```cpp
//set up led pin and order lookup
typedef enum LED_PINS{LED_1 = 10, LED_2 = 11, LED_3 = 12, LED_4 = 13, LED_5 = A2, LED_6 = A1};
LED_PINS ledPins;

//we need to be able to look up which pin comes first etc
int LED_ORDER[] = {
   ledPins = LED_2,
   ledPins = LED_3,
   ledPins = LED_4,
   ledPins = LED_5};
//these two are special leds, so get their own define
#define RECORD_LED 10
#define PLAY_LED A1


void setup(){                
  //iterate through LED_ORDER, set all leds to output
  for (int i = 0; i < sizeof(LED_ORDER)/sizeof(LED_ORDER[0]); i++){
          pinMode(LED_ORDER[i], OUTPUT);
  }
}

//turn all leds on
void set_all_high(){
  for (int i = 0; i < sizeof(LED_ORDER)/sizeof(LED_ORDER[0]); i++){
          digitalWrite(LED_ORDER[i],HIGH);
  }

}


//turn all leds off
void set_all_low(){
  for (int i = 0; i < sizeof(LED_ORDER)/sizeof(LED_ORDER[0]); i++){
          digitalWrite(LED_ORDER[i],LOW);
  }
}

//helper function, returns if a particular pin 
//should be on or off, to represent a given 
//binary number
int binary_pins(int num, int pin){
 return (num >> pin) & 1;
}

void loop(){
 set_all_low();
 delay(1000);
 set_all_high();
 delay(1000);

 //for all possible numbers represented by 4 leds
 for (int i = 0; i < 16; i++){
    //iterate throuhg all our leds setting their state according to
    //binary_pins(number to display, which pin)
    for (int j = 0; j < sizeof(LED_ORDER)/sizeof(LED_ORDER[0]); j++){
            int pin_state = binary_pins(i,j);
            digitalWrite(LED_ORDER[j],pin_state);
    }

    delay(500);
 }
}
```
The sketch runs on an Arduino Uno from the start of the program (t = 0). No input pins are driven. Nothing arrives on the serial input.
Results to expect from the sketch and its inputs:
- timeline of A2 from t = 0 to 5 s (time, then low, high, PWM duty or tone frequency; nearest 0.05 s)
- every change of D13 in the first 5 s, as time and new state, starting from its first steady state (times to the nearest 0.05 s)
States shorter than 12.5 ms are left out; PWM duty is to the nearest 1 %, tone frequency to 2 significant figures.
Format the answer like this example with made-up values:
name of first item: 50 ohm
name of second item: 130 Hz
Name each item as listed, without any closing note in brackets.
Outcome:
timeline of A2 from t = 0 to 5 s: 0 s low; 1 s high; 2 s low
every change of D13 in the first 5 s, as time and new state, starting from its first steady state: 0 s low; 1 s high; 2 s low; 4 s high
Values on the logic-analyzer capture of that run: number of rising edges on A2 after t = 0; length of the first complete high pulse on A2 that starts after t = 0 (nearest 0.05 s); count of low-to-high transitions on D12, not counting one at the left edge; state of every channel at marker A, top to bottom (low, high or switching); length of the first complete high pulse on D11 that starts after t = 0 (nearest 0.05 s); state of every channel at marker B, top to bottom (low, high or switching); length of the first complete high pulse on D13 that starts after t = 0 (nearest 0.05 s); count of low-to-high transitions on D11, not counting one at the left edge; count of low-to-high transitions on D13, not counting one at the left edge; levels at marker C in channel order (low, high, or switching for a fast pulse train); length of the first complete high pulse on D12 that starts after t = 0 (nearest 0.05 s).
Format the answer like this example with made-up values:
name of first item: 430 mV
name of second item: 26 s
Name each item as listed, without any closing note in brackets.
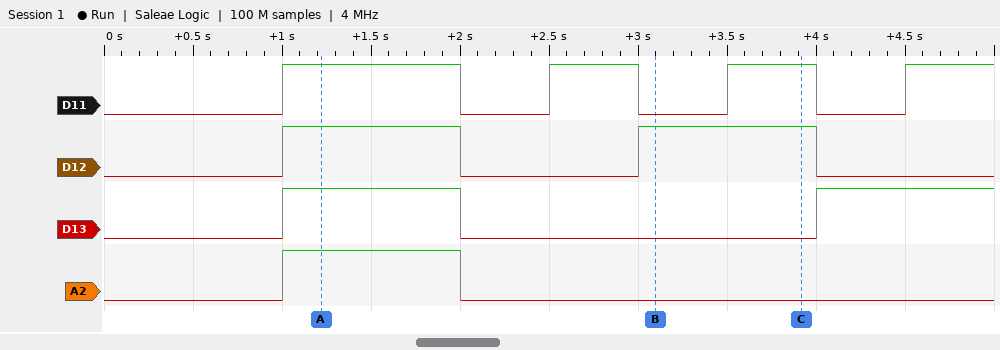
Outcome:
number of rising edges on A2 after t = 0: 1
length of the first complete high pulse on A2 that starts after t = 0: 1.00 s
count of low-to-high transitions on D12, not counting one at the left edge: 2
state of every channel at marker A, top to bottom: D11 high, D12 high, D13 high, A2 high
length of the first complete high pulse on D11 that starts after t = 0: 1.00 s
state of every channel at marker B, top to bottom: D11 low, D12 high, D13 low, A2 low
length of the first complete high pulse on D13 that starts after t = 0: 1.00 s
count of low-to-high transitions on D11, not counting one at the left edge: 4
count of low-to-high transitions on D13, not counting one at the left edge: 2
levels at marker C in channel order: D11 high, D12 high, D13 low, A2 low
length of the first complete high pulse on D12 that starts after t = 0: 1.00 s
